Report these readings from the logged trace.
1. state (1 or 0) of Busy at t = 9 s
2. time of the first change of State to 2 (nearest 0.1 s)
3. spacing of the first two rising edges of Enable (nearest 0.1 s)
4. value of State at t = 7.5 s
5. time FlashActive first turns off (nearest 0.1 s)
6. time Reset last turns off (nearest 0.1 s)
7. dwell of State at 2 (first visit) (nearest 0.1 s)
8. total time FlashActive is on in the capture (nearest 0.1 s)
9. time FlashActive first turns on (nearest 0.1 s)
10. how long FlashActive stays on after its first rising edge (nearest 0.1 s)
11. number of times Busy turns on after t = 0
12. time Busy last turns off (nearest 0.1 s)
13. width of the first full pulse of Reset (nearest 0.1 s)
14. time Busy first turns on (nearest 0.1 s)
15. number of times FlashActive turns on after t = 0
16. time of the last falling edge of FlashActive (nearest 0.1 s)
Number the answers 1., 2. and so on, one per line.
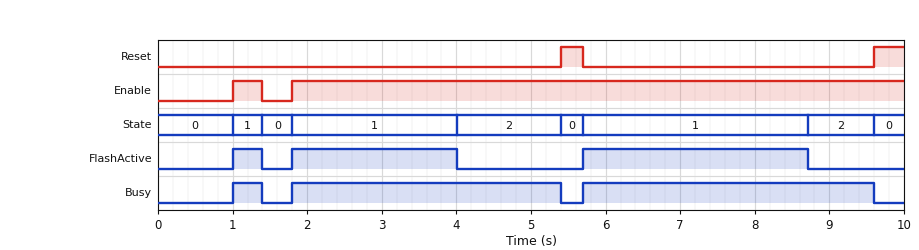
1. 1
2. 4.0 s
3. 0.8 s
4. 1
5. 1.4 s
6. 5.7 s
7. 1.4 s
8. 5.6 s
9. 1.0 s
10. 0.4 s
11. 3
12. 9.6 s
13. 0.3 s
14. 1.0 s
15. 3
16. 8.7 s
